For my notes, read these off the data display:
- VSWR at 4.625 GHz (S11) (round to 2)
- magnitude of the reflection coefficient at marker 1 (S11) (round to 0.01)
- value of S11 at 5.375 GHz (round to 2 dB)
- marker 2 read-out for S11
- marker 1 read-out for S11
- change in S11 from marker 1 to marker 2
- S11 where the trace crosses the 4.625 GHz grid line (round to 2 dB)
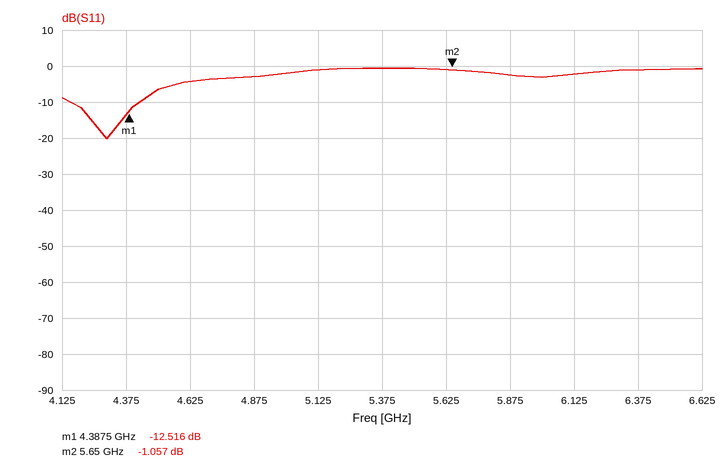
4
0.24
0 dB
-1.057 dB
-12.516 dB
11.459 dB
-4 dB
